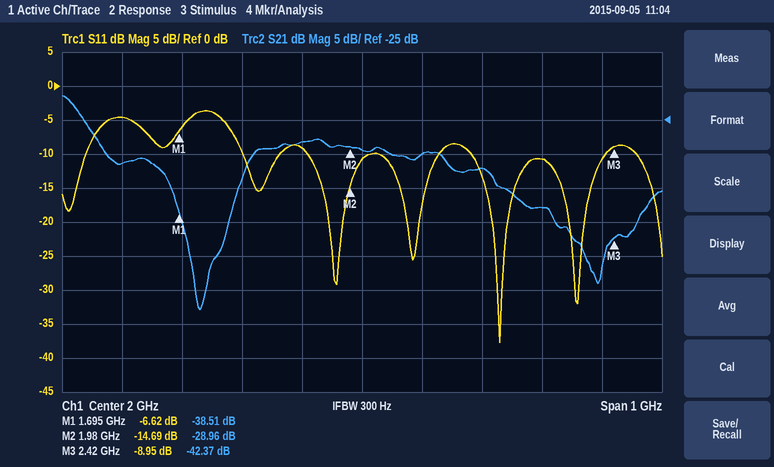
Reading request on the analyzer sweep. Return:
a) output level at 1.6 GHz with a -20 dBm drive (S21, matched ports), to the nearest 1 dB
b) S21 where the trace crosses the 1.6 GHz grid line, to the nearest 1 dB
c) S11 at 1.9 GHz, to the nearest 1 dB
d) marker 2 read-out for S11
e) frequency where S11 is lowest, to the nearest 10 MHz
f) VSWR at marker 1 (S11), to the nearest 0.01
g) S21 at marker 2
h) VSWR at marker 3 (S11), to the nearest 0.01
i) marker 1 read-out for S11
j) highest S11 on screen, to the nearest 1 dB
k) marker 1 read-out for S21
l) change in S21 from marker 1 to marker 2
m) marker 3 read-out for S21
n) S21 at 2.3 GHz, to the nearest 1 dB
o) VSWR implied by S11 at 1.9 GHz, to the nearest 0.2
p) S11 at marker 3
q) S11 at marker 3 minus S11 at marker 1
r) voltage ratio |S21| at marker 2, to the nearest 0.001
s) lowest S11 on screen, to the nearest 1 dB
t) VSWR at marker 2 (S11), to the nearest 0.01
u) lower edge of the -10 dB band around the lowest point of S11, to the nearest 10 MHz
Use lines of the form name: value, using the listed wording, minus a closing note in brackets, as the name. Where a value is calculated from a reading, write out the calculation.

output level at 1.6 GHz with a -20 dBm drive (S21, matched ports), to the nearest 1 dB: -20 dBm + (-31 dB) = -51 dBm
S21 where the trace crosses the 1.6 GHz grid line, to the nearest 1 dB: -31 dB
S11 at 1.9 GHz, to the nearest 1 dB: -9 dB
marker 2 read-out for S11: -14.69 dB
frequency where S11 is lowest, to the nearest 10 MHz: 2.23 GHz
VSWR at marker 1 (S11), to the nearest 0.01: (1 + 0.4667)/(1 − 0.4667) ≈ 2.75
S21 at marker 2: -28.96 dB
VSWR at marker 3 (S11), to the nearest 0.01: (1 + 0.3569)/(1 − 0.3569) ≈ 2.11
marker 1 read-out for S11: -6.62 dB
highest S11 on screen, to the nearest 1 dB: -4 dB
marker 1 read-out for S21: -38.51 dB
change in S21 from marker 1 to marker 2: -28.96 − (-38.51) = 9.55 dB
marker 3 read-out for S21: -42.37 dB
S21 at 2.3 GHz, to the nearest 1 dB: -38 dB
VSWR implied by S11 at 1.9 GHz, to the nearest 0.2: |Γ| = 10^(-9/20) = 0.3548; VSWR = (1 + 0.3548)/(1 − 0.3548) ≈ 2.10, so 2.0 to the nearest 0.2
S11 at marker 3: -8.95 dB
S11 at marker 3 minus S11 at marker 1: -8.95 − (-6.62) = -2.33 dB
voltage ratio |S21| at marker 2, to the nearest 0.001: 10^(-28.96/20) ≈ 0.036
lowest S11 on screen, to the nearest 1 dB: -38 dB
VSWR at marker 2 (S11), to the nearest 0.01: (1 + 0.1843)/(1 − 0.1843) ≈ 1.45
lower edge of the -10 dB band around the lowest point of S11, to the nearest 10 MHz: 2.18 GHz
